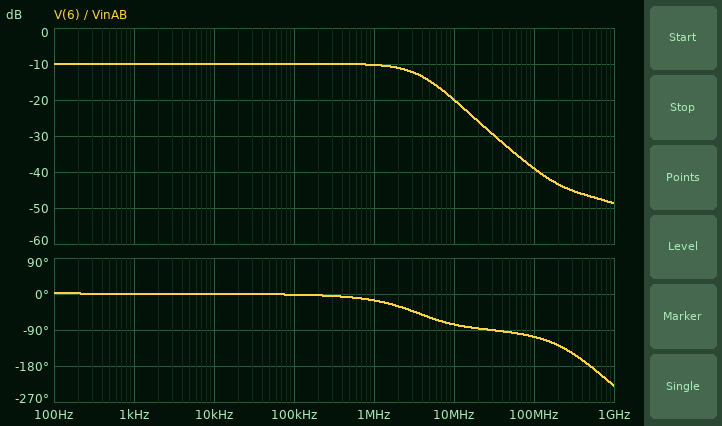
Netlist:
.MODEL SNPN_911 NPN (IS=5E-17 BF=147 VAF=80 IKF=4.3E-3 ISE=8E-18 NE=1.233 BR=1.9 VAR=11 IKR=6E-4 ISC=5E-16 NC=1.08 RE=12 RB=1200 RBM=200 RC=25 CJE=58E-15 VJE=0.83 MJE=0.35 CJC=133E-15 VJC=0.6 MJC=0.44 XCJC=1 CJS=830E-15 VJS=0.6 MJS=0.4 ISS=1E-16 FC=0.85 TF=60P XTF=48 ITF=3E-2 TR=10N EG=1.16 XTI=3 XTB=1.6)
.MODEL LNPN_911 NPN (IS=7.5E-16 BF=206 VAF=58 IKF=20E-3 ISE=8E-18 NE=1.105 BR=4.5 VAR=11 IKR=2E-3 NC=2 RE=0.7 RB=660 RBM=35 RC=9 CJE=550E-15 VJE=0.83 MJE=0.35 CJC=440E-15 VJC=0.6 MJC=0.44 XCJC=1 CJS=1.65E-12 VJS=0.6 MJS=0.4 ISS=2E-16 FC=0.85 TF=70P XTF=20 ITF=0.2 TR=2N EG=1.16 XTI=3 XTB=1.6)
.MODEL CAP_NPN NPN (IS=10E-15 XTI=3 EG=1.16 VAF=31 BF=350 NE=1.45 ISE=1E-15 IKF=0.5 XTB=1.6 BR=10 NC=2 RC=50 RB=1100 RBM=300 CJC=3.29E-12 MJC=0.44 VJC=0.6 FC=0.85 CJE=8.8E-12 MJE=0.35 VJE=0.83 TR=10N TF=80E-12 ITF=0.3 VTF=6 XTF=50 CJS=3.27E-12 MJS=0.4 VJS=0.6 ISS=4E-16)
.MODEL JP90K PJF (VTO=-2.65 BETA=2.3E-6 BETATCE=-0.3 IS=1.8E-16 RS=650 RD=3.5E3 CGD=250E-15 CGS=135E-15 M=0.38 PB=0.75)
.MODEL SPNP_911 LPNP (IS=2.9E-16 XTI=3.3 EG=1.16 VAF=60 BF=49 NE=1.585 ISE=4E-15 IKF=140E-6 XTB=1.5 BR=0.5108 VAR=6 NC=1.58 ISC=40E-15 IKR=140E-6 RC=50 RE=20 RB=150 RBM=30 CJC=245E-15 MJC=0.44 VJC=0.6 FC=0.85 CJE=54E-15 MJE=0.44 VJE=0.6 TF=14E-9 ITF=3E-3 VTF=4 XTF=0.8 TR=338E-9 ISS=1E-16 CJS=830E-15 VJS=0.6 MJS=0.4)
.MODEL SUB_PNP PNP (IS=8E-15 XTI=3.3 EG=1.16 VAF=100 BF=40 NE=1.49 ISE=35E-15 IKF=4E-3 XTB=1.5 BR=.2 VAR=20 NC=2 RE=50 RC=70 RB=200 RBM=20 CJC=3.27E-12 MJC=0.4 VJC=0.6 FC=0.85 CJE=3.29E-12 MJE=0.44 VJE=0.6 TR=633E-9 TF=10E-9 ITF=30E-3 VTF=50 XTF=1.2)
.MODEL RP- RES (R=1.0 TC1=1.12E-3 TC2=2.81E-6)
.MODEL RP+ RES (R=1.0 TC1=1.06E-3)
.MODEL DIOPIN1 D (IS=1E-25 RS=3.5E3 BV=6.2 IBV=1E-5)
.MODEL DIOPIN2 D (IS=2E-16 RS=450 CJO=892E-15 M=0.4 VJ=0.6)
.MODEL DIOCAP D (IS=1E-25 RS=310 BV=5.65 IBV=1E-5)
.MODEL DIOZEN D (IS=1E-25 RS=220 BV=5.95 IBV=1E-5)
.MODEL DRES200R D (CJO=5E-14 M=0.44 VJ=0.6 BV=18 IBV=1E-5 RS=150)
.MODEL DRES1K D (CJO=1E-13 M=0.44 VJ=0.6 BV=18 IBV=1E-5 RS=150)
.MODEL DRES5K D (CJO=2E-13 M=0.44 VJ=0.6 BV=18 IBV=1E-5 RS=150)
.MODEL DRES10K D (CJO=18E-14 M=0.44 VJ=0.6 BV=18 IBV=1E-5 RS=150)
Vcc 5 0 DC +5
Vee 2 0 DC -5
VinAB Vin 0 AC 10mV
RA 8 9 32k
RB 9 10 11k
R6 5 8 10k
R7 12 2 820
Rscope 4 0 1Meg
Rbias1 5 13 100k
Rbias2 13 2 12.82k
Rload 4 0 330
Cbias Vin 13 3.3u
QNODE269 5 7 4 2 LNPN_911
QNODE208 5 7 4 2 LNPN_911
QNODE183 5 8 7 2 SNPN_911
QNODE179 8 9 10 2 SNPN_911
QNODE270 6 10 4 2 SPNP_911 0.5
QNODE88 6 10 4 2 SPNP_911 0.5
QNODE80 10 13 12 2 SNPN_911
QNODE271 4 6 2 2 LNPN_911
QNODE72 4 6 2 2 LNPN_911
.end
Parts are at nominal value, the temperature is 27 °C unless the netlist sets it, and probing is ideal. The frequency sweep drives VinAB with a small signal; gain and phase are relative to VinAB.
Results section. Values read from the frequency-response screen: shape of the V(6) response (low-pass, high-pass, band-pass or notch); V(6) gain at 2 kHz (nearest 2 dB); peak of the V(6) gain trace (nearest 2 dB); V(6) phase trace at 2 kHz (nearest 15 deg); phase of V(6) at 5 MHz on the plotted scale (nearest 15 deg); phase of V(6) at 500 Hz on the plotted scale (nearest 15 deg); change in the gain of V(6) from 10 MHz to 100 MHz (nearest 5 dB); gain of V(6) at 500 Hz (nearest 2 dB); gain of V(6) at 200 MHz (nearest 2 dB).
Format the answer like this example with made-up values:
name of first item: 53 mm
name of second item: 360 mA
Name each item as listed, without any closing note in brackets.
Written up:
shape of the V(6) response: low-pass
V(6) gain at 2 kHz: -10 dB
peak of the V(6) gain trace: -10 dB
V(6) phase trace at 2 kHz: 0 deg
phase of V(6) at 5 MHz on the plotted scale: -60 deg
phase of V(6) at 500 Hz on the plotted scale: 0 deg
change in the gain of V(6) from 10 MHz to 100 MHz: -20 dB
gain of V(6) at 500 Hz: -10 dB
gain of V(6) at 200 MHz: -44 dB
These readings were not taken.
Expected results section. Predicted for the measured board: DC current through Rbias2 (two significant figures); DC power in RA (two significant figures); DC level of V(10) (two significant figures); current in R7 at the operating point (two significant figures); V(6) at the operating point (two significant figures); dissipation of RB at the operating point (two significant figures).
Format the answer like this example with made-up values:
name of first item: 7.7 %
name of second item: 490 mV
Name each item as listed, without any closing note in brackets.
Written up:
DC current through Rbias2: 86 µA
DC power in RA: 130 µW
DC level of V(10): 1.1 V
current in R7 at the operating point: 390 µA
V(6) at the operating point: -4.0 V
dissipation of RB at the operating point: 45 µW
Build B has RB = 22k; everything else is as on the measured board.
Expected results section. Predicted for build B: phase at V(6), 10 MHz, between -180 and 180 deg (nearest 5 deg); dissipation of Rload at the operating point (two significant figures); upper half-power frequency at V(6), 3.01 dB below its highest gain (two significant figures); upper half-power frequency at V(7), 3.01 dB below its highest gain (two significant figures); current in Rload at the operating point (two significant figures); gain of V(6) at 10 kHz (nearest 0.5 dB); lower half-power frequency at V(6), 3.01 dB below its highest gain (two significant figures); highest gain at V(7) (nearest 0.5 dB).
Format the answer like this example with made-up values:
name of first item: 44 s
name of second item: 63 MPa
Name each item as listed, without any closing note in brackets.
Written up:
phase at V(6), 10 MHz, between -180 and 180 deg: -60 deg
dissipation of Rload at the operating point: 180 µW
upper half-power frequency at V(6), 3.01 dB below its highest gain: 13 MHz
upper half-power frequency at V(7), 3.01 dB below its highest gain: 12 MHz
current in Rload at the operating point: 740 µA
gain of V(6) at 10 kHz: -4.5 dB
lower half-power frequency at V(6), 3.01 dB below its highest gain: 4.7 Hz
highest gain at V(7): 20.5 dB
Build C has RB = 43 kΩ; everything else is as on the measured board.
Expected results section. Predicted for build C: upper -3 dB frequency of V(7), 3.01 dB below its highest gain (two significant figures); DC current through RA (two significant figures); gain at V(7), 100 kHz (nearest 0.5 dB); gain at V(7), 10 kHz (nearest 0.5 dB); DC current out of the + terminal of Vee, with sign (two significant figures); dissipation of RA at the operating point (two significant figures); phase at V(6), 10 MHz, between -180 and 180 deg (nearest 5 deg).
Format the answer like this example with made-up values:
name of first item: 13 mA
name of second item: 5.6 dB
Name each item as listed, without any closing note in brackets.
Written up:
upper -3 dB frequency of V(7), 3.01 dB below its highest gain: 290 kHz
DC current through RA: 21 µA
gain at V(7), 100 kHz: 14.5 dB
gain at V(7), 10 kHz: 15.0 dB
DC current out of the + terminal of Vee, with sign: -480 µA
dissipation of RA at the operating point: 14 µW
phase at V(6), 10 MHz, between -180 and 180 deg: 140 deg
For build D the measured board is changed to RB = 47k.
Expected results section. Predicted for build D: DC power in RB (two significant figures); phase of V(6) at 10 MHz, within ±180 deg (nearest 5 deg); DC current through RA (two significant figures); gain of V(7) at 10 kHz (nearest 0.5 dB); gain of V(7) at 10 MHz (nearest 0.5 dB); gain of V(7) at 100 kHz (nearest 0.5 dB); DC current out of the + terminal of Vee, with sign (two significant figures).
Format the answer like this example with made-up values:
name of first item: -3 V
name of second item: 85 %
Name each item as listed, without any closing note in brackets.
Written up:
DC power in RB: 13 µW
phase of V(6) at 10 MHz, within ±180 deg: 140 deg
DC current through RA: 20 µA
gain of V(7) at 10 kHz: 15.0 dB
gain of V(7) at 10 MHz: -9.0 dB
gain of V(7) at 100 kHz: 14.5 dB
DC current out of the + terminal of Vee, with sign: -480 µA
